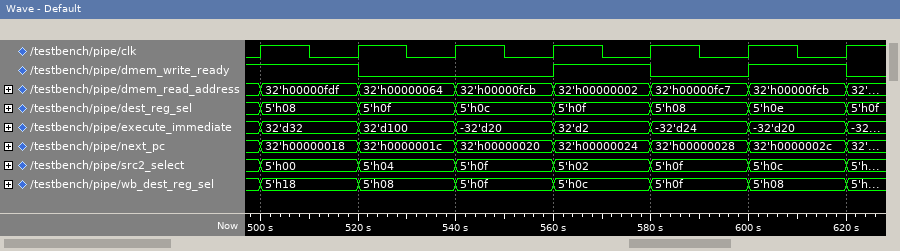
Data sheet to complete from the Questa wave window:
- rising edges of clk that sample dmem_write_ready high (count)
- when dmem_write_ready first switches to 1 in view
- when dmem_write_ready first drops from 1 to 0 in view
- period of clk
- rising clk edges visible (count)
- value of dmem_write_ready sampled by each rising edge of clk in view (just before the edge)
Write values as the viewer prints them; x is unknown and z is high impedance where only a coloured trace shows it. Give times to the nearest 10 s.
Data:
4
560 s
520 s
20 s
7
1 1 0 0 1 0 1
